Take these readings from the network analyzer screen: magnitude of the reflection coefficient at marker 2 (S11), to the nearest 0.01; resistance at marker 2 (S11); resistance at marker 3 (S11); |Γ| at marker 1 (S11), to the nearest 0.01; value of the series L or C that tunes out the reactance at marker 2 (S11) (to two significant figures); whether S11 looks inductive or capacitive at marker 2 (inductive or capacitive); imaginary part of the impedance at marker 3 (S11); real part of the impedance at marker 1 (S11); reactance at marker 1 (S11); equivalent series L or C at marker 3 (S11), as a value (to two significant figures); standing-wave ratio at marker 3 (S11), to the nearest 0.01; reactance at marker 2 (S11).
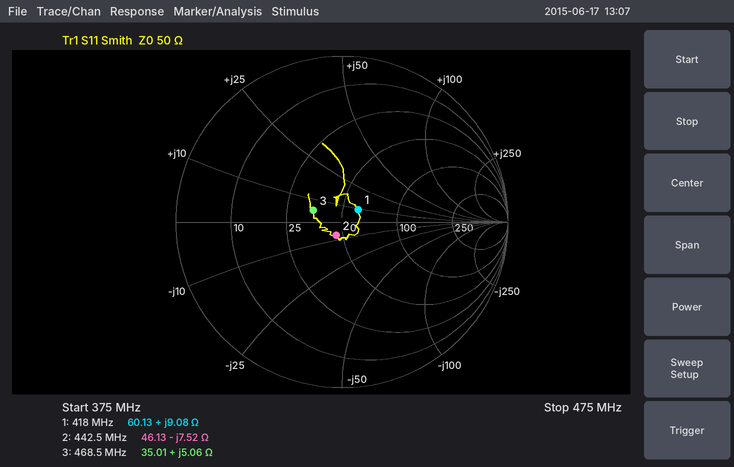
0.09
46.13 Ω
35.01 Ω
0.12
2.7 nH
capacitive
+5.06 Ω
60.13 Ω
+9.08 Ω
1.7 nH
1.46
-7.52 Ω
